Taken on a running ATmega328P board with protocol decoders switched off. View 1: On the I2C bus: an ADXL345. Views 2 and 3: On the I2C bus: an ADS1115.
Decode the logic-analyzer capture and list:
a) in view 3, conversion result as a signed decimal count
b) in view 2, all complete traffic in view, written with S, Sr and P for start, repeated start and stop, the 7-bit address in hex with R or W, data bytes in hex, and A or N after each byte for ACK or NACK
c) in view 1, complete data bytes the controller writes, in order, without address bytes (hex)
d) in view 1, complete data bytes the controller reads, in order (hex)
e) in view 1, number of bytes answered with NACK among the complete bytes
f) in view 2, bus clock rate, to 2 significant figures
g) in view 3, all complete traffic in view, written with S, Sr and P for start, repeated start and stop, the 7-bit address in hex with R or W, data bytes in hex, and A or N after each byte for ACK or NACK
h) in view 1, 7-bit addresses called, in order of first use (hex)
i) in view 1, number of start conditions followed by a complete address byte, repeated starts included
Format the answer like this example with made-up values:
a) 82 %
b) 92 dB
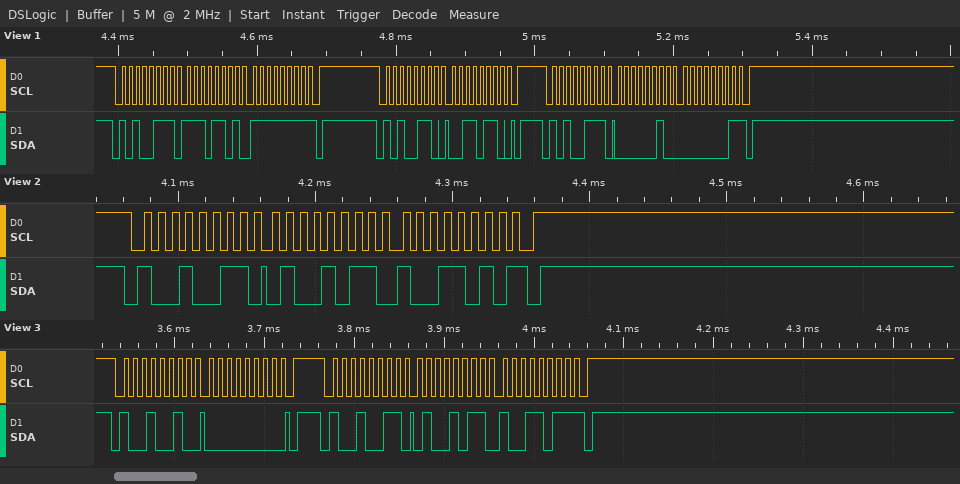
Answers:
a) 19355
b) S 49R A 4B A 9A N P
c) 36
d) ED FF 02 01
e) 2
f) 100 kHz
g) S 49W A 00 A P S 49R A 4B A 9B N P
h) 0x53
i) 3
